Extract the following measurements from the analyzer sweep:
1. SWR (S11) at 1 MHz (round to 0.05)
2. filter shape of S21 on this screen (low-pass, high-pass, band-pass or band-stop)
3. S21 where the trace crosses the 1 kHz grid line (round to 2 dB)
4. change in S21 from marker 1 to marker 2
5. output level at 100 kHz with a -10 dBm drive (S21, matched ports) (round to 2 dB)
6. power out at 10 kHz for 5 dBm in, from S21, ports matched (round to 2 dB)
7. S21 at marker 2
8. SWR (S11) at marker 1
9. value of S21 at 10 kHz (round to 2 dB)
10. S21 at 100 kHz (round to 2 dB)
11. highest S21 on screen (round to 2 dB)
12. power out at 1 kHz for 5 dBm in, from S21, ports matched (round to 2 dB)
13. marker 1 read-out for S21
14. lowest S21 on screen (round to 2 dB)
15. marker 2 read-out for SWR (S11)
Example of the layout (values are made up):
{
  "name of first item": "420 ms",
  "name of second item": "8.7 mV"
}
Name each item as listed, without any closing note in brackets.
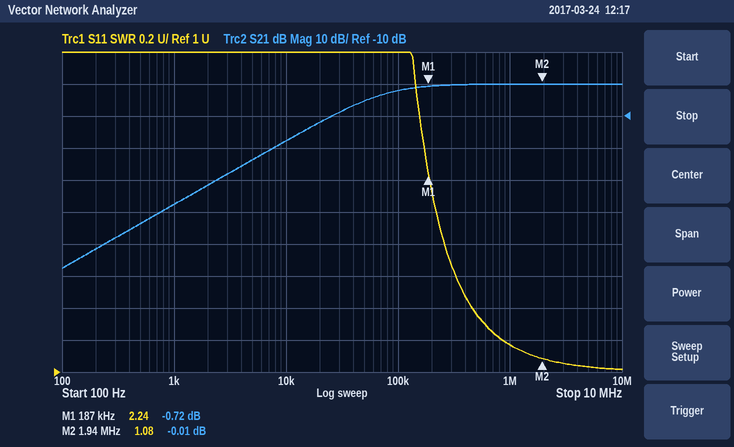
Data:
{
  "SWR (S11) at 1 MHz": "1.15",
  "filter shape of S21 on this screen": "high-pass",
  "S21 where the trace crosses the 1 kHz grid line": "-38 dB",
  "change in S21 from marker 1 to marker 2": "0.71 dB",
  "output level at 100 kHz with a -10 dBm drive (S21, matched ports)": "-12 dBm",
  "power out at 10 kHz for 5 dBm in, from S21, ports matched": "-12 dBm",
  "S21 at marker 2": "-0.01 dB",
  "SWR (S11) at marker 1": "2.24",
  "value of S21 at 10 kHz": "-18 dB",
  "S21 at 100 kHz": "-2 dB",
  "highest S21 on screen": "0 dB",
  "power out at 1 kHz for 5 dBm in, from S21, ports matched": "-32 dBm",
  "marker 1 read-out for S21": "-0.72 dB",
  "lowest S21 on screen": "-58 dB",
  "marker 2 read-out for SWR": "1.08"
}
